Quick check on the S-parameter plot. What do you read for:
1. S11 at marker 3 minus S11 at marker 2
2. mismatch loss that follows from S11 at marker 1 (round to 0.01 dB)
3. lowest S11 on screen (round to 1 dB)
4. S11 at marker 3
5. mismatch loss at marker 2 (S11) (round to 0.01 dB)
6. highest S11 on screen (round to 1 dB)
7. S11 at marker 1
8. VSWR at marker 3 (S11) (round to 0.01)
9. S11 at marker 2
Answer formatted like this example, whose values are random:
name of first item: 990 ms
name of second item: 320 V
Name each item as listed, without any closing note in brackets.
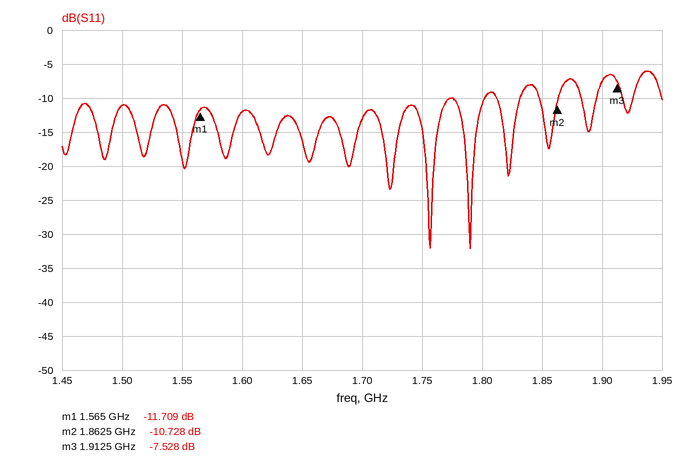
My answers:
S11 at marker 3 minus S11 at marker 2: 3.200 dB
mismatch loss that follows from S11 at marker 1: 0.30 dB
lowest S11 on screen: -32 dB
S11 at marker 3: -7.528 dB
mismatch loss at marker 2 (S11): 0.38 dB
highest S11 on screen: -6 dB
S11 at marker 1: -11.709 dB
VSWR at marker 3 (S11): 2.45
S11 at marker 2: -10.728 dB
